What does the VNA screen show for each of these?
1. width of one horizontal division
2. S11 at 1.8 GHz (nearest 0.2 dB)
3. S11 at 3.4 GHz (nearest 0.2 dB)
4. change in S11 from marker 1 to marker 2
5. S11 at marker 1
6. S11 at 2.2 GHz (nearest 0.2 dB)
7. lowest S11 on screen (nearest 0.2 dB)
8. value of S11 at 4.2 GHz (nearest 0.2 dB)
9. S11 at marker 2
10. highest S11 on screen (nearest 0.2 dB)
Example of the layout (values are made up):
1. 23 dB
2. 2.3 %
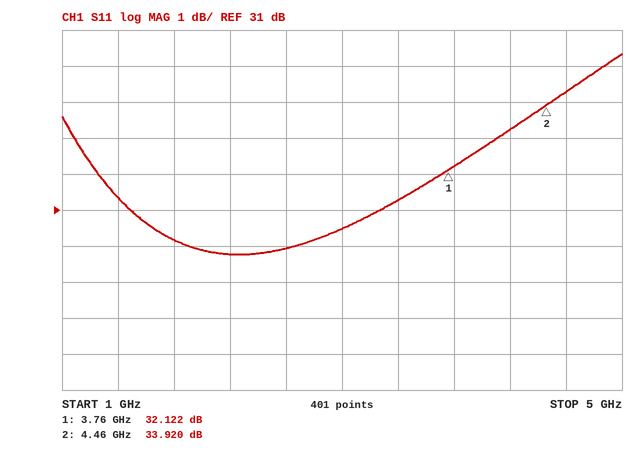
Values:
1. 400 MHz
2. 30.2 dB
3. 31.2 dB
4. 1.798 dB
5. 32.122 dB
6. 29.8 dB
7. 29.8 dB
8. 33.2 dB
9. 33.920 dB
10. 35.4 dB
